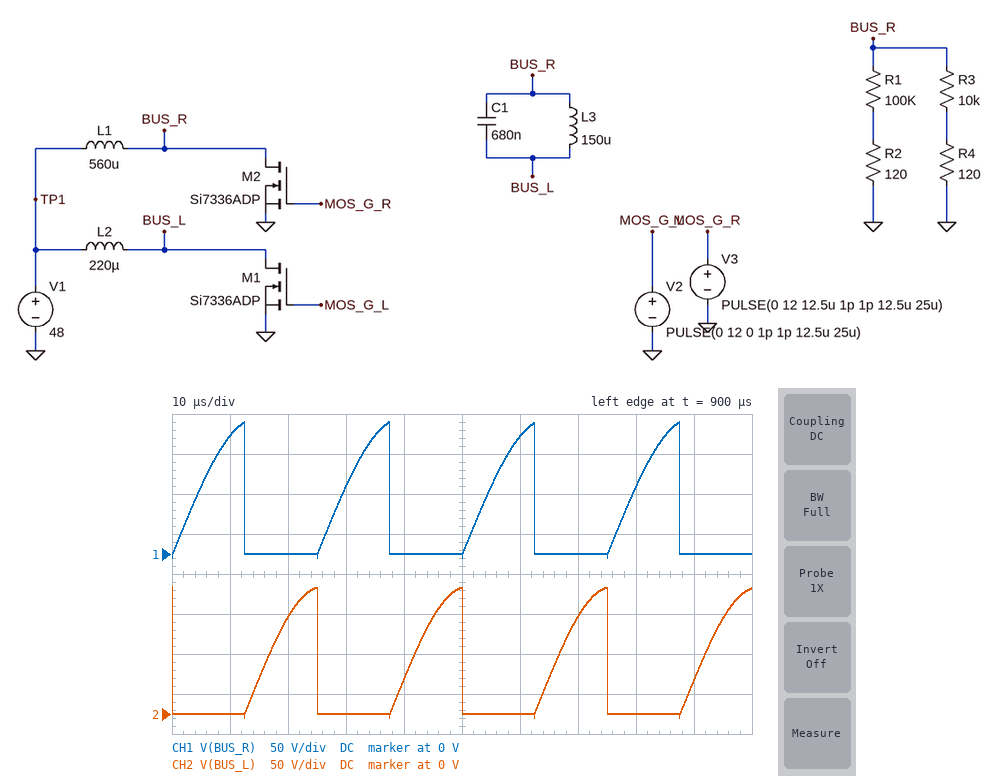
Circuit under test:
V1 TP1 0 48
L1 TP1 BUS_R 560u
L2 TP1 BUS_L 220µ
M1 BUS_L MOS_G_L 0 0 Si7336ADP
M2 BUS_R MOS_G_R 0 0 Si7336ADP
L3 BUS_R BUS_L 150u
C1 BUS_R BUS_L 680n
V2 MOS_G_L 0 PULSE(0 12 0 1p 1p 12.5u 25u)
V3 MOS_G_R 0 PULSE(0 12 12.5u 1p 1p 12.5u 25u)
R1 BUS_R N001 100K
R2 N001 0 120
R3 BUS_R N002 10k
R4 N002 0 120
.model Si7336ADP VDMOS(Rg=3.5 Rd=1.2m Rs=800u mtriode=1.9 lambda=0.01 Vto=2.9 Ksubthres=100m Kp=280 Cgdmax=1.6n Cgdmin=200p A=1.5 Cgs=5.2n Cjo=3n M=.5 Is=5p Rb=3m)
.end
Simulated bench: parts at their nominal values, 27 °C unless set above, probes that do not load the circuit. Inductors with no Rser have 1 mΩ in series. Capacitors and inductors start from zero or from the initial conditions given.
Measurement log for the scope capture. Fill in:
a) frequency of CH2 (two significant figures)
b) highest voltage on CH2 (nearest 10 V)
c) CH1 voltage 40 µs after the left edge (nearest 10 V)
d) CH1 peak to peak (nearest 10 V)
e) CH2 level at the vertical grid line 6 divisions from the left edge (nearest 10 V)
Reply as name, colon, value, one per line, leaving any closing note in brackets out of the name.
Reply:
frequency of CH2: 40 kHz
highest voltage on CH2: 160 V
CH1 voltage 40 µs after the left edge: 0 V
CH1 peak to peak: 170 V
CH2 level at the vertical grid line 6 divisions from the left edge: 0 V
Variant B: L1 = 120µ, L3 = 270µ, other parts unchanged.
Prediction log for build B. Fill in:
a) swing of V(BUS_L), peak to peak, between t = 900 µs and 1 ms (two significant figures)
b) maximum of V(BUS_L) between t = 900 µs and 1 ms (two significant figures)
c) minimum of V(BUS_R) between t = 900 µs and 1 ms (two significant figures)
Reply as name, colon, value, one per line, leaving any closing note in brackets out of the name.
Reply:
swing of V(BUS_L), peak to peak, between t = 900 µs and 1 ms: 180 V
maximum of V(BUS_L) between t = 900 µs and 1 ms: 170 V
minimum of V(BUS_R) between t = 900 µs and 1 ms: -5.4 V
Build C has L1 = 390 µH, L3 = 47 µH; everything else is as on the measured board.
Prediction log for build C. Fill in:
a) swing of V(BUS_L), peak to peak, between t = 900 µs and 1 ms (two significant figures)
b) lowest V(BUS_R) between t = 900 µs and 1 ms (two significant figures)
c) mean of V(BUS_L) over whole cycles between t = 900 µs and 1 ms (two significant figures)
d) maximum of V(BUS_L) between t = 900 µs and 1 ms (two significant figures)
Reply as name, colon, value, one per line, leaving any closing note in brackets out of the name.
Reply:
swing of V(BUS_L), peak to peak, between t = 900 µs and 1 ms: 140 V
lowest V(BUS_R) between t = 900 µs and 1 ms: -4.6 V
mean of V(BUS_L) over whole cycles between t = 900 µs and 1 ms: 48 V
maximum of V(BUS_L) between t = 900 µs and 1 ms: 130 V
